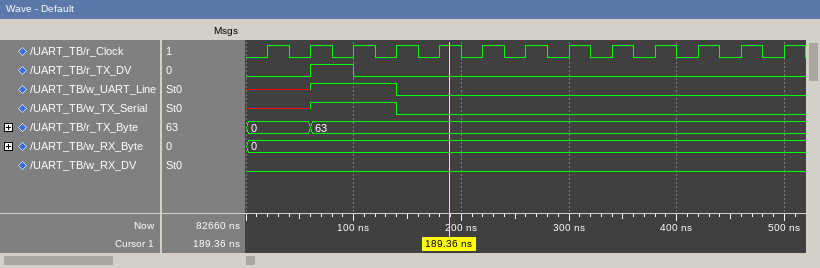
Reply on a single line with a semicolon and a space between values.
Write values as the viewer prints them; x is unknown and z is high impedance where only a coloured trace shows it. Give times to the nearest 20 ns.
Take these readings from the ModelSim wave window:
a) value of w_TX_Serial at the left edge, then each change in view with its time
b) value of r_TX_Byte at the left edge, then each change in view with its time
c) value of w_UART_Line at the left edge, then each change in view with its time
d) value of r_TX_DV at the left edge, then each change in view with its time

x, 1 at 60 ns, 0 at 140 ns; 0, 63 at 60 ns; x, 1 at 60 ns, 0 at 140 ns; 0, 1 at 60 ns, 0 at 100 ns
